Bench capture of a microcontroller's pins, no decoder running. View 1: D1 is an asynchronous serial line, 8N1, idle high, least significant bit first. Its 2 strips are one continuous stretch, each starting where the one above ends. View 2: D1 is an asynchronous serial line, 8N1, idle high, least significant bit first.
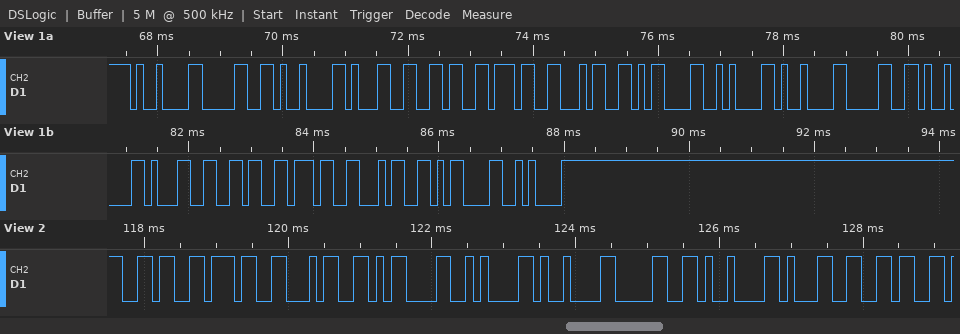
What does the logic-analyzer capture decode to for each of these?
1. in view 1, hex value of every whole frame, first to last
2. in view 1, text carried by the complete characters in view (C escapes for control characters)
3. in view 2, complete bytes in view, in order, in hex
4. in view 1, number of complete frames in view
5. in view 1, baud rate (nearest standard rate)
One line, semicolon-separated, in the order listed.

0x09 0x30 0x09 0x31 0x36 0x37 0x34 0x0D 0x0A 0x09 0x30 0x09 0x31 0x36 0x37 0x34 0x0D 0x0A; "\t0\t1674\r\n\t0\t1674\r\n"; 36 37 34 0D 0A 09 30 09 31 36; 18; 9600 baud
